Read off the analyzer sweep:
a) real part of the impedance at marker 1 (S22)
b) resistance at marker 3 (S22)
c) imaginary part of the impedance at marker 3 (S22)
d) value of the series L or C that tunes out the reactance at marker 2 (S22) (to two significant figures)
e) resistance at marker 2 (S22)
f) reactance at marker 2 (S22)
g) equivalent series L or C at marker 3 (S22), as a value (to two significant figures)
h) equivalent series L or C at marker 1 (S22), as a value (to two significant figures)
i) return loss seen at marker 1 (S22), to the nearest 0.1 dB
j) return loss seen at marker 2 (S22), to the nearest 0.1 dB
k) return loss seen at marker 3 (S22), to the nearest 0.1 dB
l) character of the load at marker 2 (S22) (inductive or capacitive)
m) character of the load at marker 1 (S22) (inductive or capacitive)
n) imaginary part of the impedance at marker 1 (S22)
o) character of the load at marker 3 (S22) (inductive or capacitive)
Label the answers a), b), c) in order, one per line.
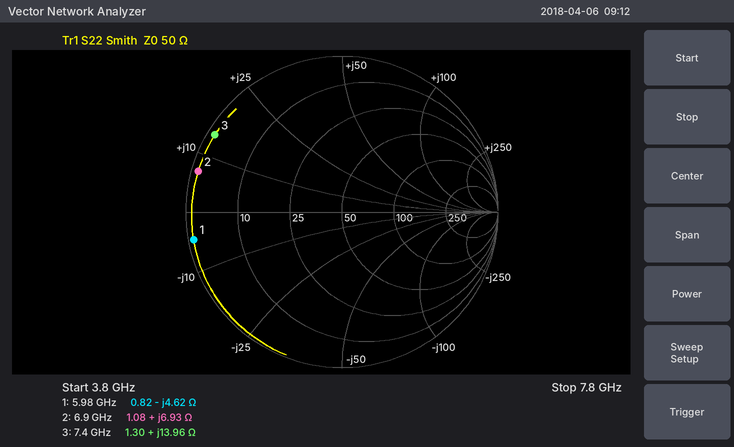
a) 0.82 Ω
b) 1.30 Ω
c) +13.96 Ω
d) 3.3 pF
e) 1.08 Ω
f) +6.93 Ω
g) 300 pH
h) 5.8 pF
i) 0.3 dB
j) 0.4 dB
k) 0.4 dB
l) inductive
m) capacitive
n) -4.62 Ω
o) inductive
